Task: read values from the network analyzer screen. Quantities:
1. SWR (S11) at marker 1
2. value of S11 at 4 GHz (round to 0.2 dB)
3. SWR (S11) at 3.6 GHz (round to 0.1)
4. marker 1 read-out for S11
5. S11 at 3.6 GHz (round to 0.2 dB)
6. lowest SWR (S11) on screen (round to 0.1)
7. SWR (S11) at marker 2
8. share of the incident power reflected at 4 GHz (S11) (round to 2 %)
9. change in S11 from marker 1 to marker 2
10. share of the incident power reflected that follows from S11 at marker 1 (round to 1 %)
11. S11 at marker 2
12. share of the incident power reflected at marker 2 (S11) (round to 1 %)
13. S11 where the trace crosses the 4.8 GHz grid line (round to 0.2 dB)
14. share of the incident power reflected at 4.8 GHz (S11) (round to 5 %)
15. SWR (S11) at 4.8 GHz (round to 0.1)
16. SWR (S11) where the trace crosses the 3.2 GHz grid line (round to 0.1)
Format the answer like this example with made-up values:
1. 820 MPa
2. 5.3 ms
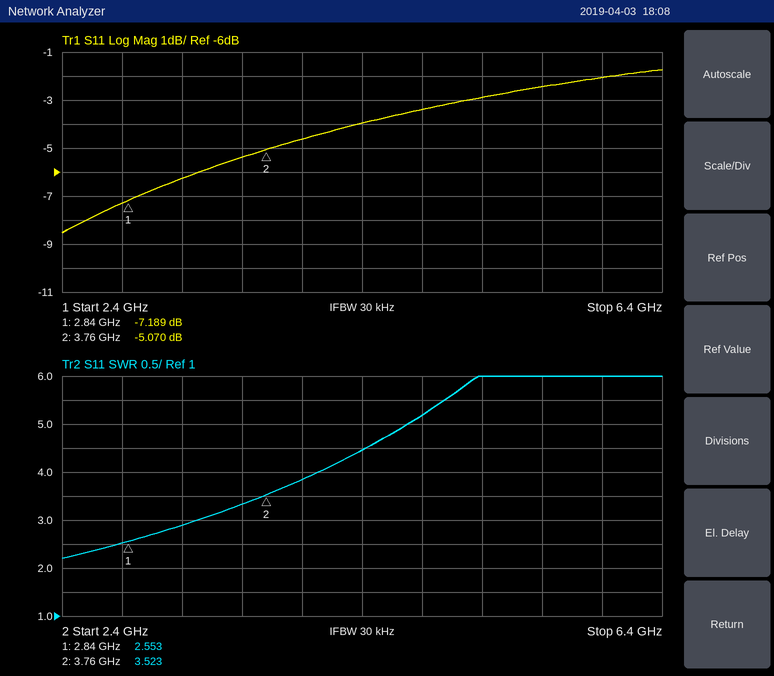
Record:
1. 2.553
2. -4.6 dB
3. 3.3
4. -7.189 dB
5. -5.4 dB
6. 2.2
7. 3.523
8. 34 %
9. 2.119 dB
10. 19 %
11. -5.070 dB
12. 31 %
13. -3.4 dB
14. 45 %
15. 5.2
16. 2.9
